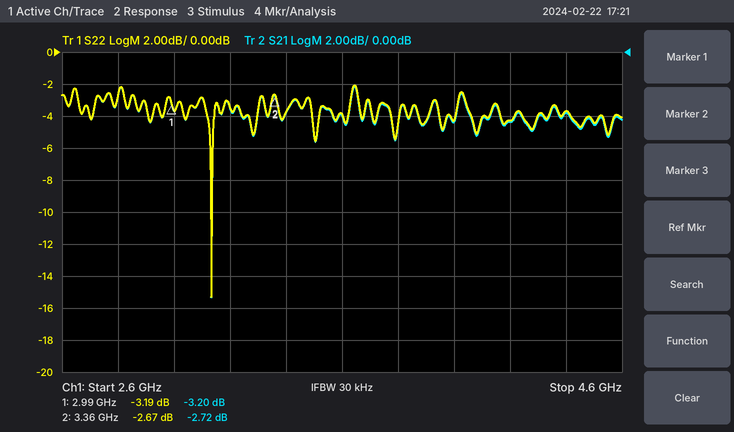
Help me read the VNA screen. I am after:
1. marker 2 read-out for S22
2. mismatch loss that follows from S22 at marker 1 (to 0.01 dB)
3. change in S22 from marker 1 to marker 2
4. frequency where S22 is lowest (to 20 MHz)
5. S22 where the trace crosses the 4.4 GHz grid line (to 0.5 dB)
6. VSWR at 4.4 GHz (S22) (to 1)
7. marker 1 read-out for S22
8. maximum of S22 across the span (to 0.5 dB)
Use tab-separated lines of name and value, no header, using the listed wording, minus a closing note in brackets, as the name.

marker 2 read-out for S22	-2.67 dB
mismatch loss that follows from S22 at marker 1	2.84 dB
change in S22 from marker 1 to marker 2	0.52 dB
frequency where S22 is lowest	3.14 GHz
S22 where the trace crosses the 4.4 GHz grid line	-3.5 dB
VSWR at 4.4 GHz (S22)	5
marker 1 read-out for S22	-3.19 dB
maximum of S22 across the span	-2.0 dB
